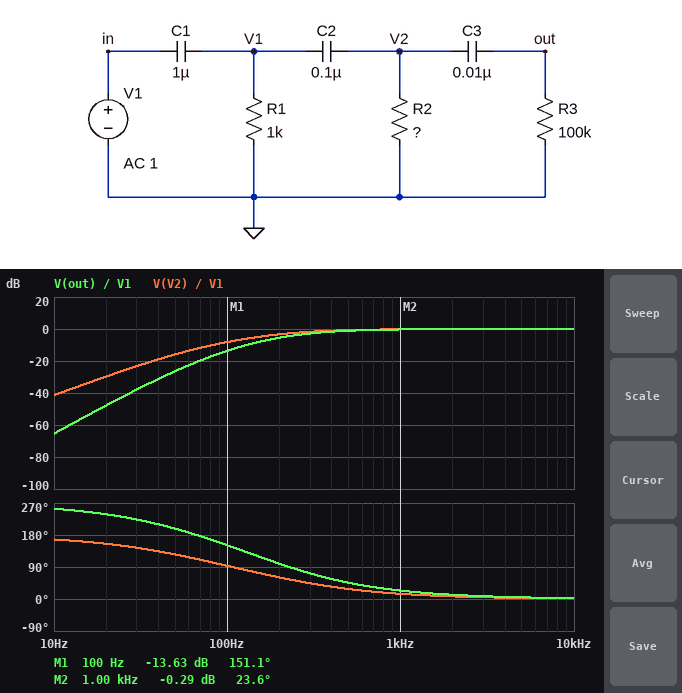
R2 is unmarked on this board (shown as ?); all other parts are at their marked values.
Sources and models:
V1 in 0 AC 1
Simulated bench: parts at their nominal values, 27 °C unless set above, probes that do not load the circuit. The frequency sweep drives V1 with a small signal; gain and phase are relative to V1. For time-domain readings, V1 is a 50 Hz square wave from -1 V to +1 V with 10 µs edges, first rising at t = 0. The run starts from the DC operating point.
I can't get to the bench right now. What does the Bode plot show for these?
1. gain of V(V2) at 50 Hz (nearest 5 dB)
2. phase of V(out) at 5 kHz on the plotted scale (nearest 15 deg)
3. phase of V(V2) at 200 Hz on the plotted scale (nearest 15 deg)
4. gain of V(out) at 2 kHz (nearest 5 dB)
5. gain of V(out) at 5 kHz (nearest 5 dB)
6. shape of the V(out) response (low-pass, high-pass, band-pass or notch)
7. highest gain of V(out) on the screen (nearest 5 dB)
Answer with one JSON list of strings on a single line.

["-15 dB", "0 deg", "60 deg", "0 dB", "0 dB", "high-pass", "0 dB"]
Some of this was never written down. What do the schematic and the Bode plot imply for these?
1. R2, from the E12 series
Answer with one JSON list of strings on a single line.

["22 kΩ"]
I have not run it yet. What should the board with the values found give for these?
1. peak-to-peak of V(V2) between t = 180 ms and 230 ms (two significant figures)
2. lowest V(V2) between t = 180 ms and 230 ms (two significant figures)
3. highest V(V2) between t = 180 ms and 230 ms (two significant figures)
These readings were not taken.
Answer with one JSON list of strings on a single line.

["4.0 V", "-2.0 V", "2.0 V"]
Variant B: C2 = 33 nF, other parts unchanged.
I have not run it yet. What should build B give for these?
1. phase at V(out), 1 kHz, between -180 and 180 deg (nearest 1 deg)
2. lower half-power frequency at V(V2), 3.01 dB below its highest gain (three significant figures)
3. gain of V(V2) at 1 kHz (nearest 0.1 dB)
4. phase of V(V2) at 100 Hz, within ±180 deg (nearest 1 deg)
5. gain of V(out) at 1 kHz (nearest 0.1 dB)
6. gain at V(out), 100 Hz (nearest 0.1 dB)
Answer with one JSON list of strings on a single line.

["33 deg", "360 Hz", "-0.5 dB", "120 deg", "-0.6 dB", "-19.5 dB"]
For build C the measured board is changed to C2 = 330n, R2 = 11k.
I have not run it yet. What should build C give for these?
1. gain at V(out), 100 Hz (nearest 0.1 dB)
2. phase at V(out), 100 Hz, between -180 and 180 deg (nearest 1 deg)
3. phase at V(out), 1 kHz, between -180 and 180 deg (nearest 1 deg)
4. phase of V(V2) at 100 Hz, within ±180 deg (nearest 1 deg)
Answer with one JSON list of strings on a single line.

["-12.5 dB", "140 deg", "22 deg", "82 deg"]
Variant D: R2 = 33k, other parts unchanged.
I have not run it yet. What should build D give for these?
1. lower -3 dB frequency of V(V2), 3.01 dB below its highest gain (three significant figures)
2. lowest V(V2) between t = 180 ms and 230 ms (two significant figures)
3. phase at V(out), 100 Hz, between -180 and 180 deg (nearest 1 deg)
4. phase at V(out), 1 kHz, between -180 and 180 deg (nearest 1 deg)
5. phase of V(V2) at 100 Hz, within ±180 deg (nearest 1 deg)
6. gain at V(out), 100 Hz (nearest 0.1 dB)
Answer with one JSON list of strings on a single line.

["197 Hz", "-2.0 V", "142 deg", "22 deg", "84 deg", "-12.7 dB"]
